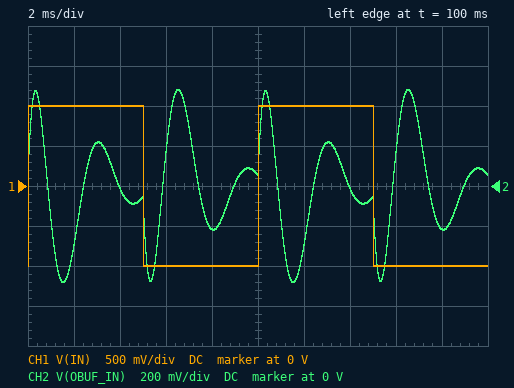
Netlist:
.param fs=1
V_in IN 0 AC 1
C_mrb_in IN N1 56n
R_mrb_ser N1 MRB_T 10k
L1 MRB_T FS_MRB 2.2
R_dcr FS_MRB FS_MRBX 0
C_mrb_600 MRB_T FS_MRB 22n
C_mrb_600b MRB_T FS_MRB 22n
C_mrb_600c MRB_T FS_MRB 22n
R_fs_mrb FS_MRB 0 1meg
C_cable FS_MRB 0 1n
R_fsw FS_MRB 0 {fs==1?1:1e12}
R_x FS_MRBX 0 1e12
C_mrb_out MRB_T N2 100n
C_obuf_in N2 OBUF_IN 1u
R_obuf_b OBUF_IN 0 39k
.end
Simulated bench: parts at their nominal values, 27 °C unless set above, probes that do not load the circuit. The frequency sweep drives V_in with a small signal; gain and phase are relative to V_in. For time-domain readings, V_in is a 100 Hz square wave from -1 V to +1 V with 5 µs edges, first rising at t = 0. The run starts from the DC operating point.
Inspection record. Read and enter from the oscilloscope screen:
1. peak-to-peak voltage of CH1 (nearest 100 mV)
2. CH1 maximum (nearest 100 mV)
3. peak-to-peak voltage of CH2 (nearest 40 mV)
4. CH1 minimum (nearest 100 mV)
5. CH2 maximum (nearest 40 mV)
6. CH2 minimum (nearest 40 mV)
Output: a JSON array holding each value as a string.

["2.0 V", "1.0 V", "960 mV", "-1.0 V", "480 mV", "-480 mV"]
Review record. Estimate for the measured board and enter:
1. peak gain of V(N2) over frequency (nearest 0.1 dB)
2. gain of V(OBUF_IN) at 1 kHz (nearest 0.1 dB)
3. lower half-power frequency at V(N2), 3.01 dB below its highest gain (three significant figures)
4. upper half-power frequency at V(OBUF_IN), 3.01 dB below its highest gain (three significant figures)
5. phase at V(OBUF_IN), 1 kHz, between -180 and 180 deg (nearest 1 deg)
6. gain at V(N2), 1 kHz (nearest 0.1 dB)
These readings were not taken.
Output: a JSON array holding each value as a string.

["-0.9 dB", "-12.1 dB", "286 Hz", "475 Hz", "-54 deg", "-12.1 dB"]
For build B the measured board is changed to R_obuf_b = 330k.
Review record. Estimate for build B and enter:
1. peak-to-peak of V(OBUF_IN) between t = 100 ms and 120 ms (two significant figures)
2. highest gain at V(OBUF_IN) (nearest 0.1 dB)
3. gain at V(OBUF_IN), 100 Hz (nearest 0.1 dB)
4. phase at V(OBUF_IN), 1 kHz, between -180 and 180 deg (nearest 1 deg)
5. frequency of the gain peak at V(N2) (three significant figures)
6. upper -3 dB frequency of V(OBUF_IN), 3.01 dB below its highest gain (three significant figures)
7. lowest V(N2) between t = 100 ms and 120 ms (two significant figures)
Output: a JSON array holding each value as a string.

["1.1 V", "1.7 dB", "-25.9 dB", "-59 deg", "359 Hz", "441 Hz", "-540 mV"]
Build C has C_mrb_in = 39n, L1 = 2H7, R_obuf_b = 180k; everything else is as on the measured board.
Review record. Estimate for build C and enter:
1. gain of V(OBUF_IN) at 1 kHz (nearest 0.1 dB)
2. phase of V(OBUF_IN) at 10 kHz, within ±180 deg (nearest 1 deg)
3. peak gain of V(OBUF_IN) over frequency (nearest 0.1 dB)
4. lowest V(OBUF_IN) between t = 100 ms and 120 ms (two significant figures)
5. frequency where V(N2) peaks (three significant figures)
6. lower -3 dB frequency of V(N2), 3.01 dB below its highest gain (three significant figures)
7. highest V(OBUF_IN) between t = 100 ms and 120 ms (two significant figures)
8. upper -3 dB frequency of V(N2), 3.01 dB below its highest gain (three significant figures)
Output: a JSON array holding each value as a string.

["-12.7 dB", "-86 deg", "3.0 dB", "-670 mV", "320 Hz", "284 Hz", "670 mV", "370 Hz"]
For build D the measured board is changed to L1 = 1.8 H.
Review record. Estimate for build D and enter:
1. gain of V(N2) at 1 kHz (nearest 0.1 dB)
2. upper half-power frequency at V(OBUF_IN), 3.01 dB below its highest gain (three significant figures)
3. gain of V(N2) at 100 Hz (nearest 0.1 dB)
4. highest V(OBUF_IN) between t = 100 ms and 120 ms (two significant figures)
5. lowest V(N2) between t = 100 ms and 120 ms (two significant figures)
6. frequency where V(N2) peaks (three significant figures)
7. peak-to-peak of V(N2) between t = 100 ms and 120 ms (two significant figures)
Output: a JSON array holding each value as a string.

["-11.8 dB", "529 Hz", "-28.5 dB", "430 mV", "-430 mV", "402 Hz", "860 mV"]
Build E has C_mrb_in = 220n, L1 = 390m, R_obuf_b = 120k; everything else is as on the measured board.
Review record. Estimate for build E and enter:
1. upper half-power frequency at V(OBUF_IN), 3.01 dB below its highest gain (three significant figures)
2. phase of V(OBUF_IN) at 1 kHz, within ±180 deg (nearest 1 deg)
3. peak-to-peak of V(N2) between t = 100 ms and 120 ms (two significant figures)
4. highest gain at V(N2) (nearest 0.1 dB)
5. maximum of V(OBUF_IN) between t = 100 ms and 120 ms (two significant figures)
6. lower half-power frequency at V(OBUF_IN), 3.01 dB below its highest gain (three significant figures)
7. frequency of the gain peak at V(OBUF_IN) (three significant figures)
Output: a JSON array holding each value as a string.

["1.12 kHz", "-2 deg", "750 mV", "-0.7 dB", "370 mV", "862 Hz", "983 Hz"]
